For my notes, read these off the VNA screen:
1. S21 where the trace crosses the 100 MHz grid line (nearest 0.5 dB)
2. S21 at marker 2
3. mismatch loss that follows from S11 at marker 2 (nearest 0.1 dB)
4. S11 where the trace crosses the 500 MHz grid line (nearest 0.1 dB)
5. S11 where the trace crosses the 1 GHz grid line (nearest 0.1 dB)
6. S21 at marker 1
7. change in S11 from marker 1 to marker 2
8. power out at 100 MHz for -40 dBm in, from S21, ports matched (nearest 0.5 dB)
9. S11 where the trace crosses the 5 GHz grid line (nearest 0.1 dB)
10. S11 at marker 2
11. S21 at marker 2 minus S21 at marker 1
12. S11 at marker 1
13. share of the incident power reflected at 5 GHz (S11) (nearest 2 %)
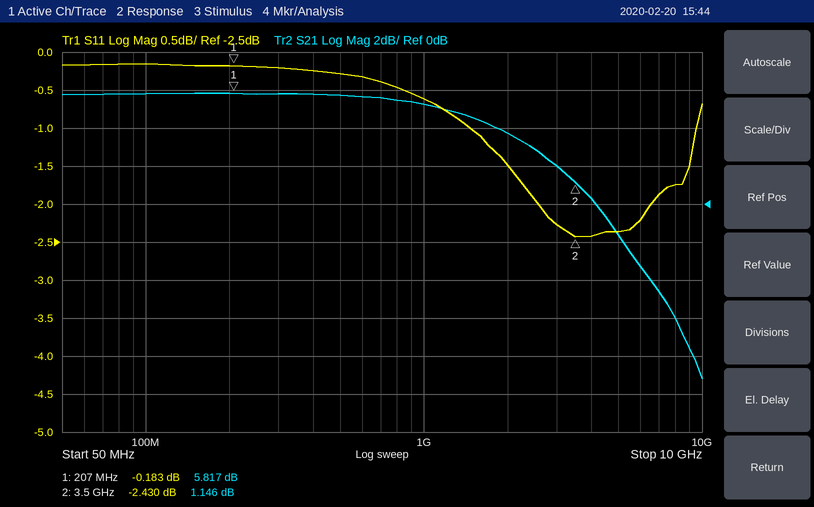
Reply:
6.0 dB
1.146 dB
3.7 dB
-0.3 dB
-0.6 dB
5.817 dB
-2.247 dB
-34.0 dBm
-2.4 dB
-2.430 dB
-4.671 dB
-0.183 dB
58 %
